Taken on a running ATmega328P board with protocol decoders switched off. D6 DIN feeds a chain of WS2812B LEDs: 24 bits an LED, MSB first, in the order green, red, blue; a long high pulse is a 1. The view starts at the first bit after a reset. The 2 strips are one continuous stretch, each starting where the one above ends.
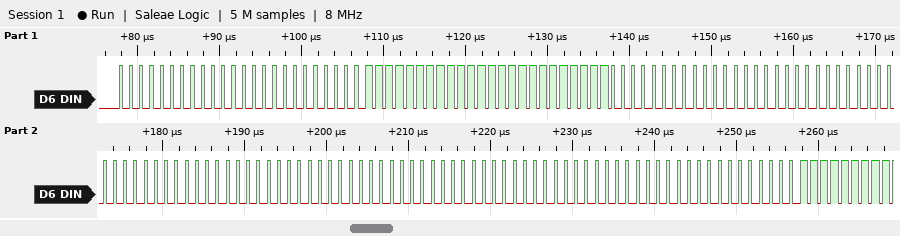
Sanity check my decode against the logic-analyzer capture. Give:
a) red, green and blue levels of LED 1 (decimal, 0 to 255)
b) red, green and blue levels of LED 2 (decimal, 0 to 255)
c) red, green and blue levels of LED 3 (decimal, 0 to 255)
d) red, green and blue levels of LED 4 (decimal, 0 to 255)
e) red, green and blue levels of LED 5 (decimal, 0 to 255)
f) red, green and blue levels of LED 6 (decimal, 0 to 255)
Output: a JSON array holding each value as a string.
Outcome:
["0, 0, 0", "255, 255, 255", "0, 0, 0", "0, 0, 0", "0, 0, 0", "0, 0, 0"]
